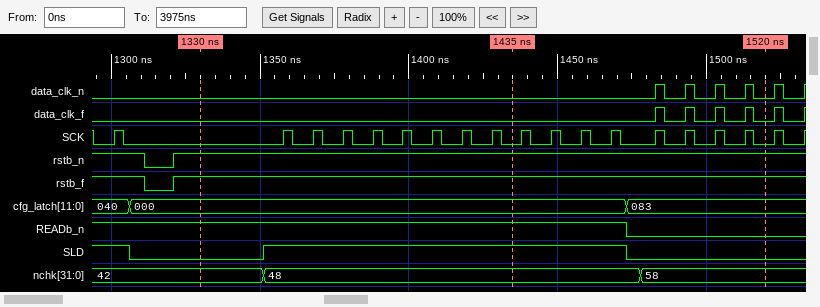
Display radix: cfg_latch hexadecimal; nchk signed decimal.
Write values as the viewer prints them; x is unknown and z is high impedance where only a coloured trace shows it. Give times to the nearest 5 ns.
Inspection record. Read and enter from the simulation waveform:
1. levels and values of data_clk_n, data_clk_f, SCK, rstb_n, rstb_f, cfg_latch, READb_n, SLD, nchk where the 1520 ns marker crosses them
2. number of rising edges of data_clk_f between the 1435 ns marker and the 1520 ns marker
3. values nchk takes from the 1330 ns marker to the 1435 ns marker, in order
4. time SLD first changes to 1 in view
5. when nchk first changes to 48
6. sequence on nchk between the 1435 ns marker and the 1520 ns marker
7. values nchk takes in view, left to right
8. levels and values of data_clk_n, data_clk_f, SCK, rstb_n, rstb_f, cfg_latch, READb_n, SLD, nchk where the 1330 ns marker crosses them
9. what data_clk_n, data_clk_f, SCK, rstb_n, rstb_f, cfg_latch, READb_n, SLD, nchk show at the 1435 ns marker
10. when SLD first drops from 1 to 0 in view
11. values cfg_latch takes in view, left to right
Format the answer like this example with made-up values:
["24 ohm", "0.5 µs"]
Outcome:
["data_clk_n=0, data_clk_f=0, SCK=0, rstb_n=1, rstb_f=1, cfg_latch=083, READb_n=0, SLD=0, nchk=58", "4", "42, 48", "1350 ns", "1350 ns", "48, 58", "42, 48, 58", "data_clk_n=0, data_clk_f=0, SCK=0, rstb_n=1, rstb_f=1, cfg_latch=000, READb_n=1, SLD=0, nchk=42", "data_clk_n=0, data_clk_f=0, SCK=0, rstb_n=1, rstb_f=1, cfg_latch=000, READb_n=1, SLD=1, nchk=48", "1305 ns", "040, 000, 083"]
